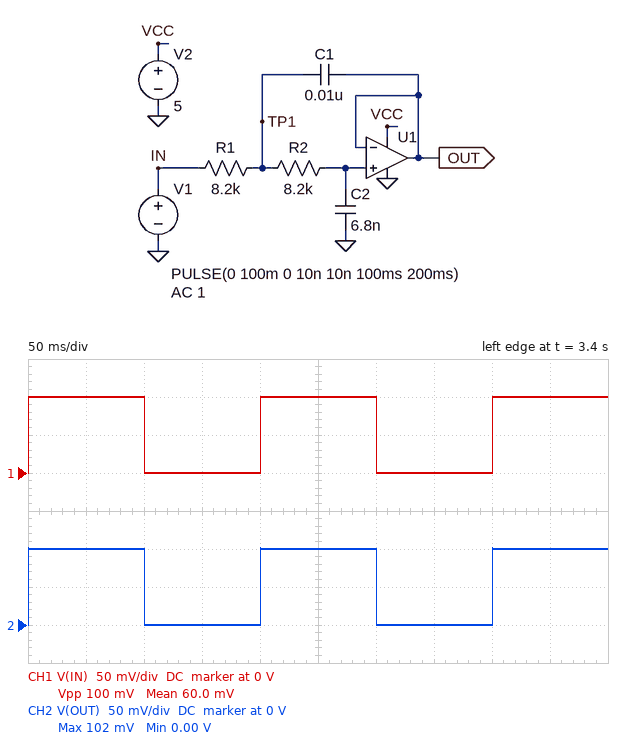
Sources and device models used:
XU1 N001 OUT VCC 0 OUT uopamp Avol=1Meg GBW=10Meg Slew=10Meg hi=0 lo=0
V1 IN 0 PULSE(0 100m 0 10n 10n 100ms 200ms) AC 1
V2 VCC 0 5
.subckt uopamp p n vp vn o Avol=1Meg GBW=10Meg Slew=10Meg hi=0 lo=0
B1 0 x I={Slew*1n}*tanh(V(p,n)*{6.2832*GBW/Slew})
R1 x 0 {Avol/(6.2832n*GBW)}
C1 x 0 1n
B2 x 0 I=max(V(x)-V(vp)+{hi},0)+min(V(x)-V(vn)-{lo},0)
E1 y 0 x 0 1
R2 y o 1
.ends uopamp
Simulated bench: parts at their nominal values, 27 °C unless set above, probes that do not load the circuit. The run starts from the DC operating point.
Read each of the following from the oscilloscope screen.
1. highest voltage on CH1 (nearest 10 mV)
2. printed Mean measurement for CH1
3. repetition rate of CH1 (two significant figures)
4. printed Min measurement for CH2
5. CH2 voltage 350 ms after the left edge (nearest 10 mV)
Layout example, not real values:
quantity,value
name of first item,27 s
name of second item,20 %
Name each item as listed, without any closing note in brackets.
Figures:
quantity,value
highest voltage on CH1,100 mV
printed Mean measurement for CH1,60.0 mV
repetition rate of CH1,5.0 Hz
printed Min measurement for CH2,0.00 V
CH2 voltage 350 ms after the left edge,0 V
